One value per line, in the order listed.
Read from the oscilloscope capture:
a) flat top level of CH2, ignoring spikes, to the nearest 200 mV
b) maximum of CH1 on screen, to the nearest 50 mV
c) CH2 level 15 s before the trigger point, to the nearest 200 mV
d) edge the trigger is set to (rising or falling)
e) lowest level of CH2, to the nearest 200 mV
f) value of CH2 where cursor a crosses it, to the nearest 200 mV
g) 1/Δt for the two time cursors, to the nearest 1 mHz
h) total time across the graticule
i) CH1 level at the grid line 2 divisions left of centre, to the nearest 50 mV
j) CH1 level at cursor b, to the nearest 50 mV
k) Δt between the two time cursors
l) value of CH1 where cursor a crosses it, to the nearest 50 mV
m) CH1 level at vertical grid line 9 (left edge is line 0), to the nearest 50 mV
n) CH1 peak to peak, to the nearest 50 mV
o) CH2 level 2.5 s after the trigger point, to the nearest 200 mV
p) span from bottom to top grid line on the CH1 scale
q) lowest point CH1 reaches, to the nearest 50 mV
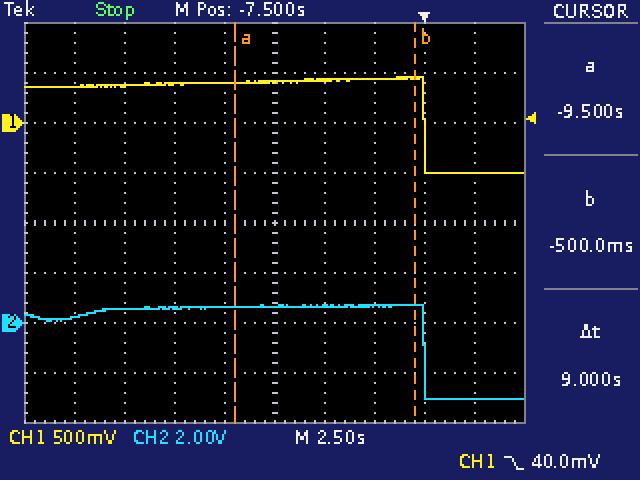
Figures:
600 mV
450 mV
600 mV
falling
-3.0 V
600 mV
111 mHz
25 s
400 mV
450 mV
9 s
400 mV
-500 mV
950 mV
-3.0 V
4 V
-500 mV
